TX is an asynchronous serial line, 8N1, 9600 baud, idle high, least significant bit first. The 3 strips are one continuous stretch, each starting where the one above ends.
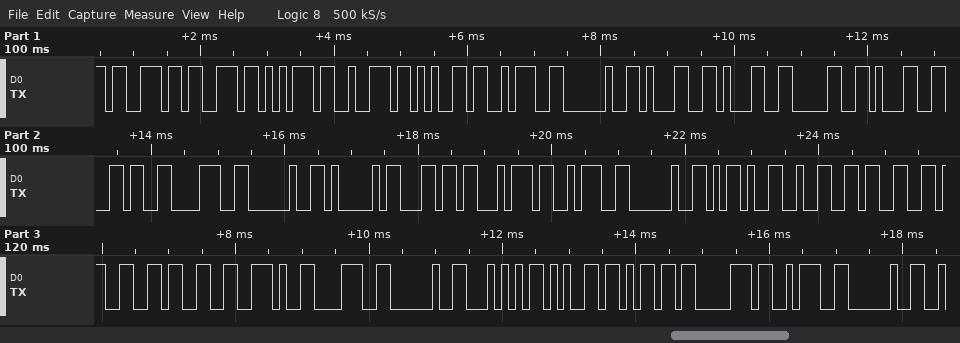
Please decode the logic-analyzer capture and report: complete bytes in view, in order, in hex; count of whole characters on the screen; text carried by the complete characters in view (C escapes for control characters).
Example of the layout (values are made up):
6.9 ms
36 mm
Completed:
0x73 0x73 0x75 0x72 0x65 0x3A 0x20 0x31 0x31 0x30 0x31 0x36 0x38 0x20 0x41 0x6C 0x74 0x3A 0x20 0x2D 0x32 0x33 0x33 0x33 0x2E 0x38 0x20 0x54 0x65 0x6D 0x70 0x3A 0x20
33
"ssure: 110168 Alt: -2333.8 Temp: "
